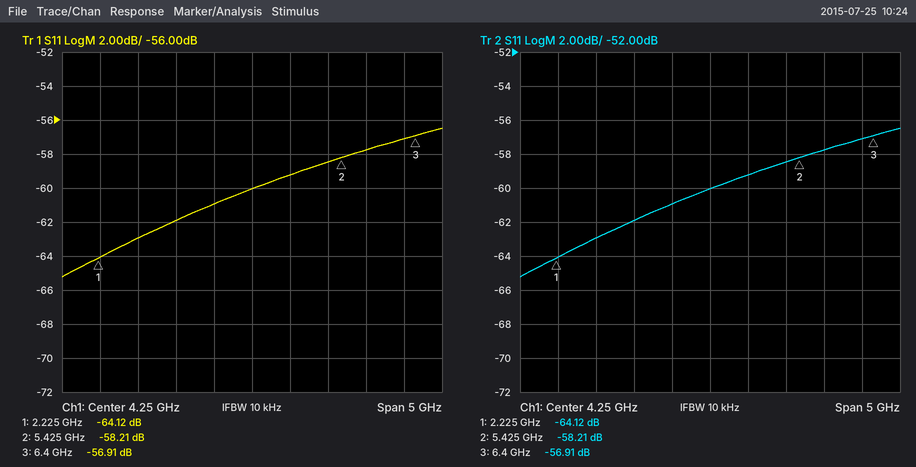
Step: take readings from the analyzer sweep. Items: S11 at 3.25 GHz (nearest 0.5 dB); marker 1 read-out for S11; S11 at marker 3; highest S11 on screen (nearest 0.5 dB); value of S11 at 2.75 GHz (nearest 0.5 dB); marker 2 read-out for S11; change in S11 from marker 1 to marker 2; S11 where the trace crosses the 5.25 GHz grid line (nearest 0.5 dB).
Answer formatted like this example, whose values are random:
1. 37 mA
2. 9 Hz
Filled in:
1. -62.0 dB
2. -64.12 dB
3. -56.91 dB
4. -56.5 dB
5. -63.0 dB
6. -58.21 dB
7. 5.91 dB
8. -58.5 dB
